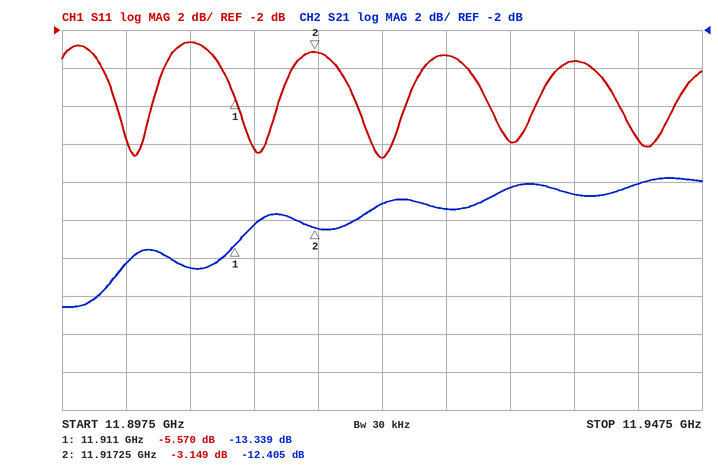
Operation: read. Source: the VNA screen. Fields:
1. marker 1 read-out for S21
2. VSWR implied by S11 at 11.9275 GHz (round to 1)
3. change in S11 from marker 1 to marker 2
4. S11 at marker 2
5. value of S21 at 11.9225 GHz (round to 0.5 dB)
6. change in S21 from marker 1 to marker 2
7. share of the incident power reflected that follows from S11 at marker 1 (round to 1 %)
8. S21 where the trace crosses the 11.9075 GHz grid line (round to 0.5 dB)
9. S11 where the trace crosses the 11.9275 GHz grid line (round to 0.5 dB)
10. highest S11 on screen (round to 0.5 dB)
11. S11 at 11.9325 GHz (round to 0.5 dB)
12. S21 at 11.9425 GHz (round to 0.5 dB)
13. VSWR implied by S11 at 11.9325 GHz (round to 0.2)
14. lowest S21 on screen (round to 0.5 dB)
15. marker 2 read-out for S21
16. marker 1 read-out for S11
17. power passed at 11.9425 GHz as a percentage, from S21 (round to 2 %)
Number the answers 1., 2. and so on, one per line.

1. -13.339 dB
2. 5
3. 2.421 dB
4. -3.149 dB
5. -11.0 dB
6. 0.934 dB
7. 28 %
8. -14.5 dB
9. -3.5 dB
10. -2.5 dB
11. -8.0 dB
12. -10.0 dB
13. 2.4
14. -16.5 dB
15. -12.405 dB
16. -5.570 dB
17. 10 %
